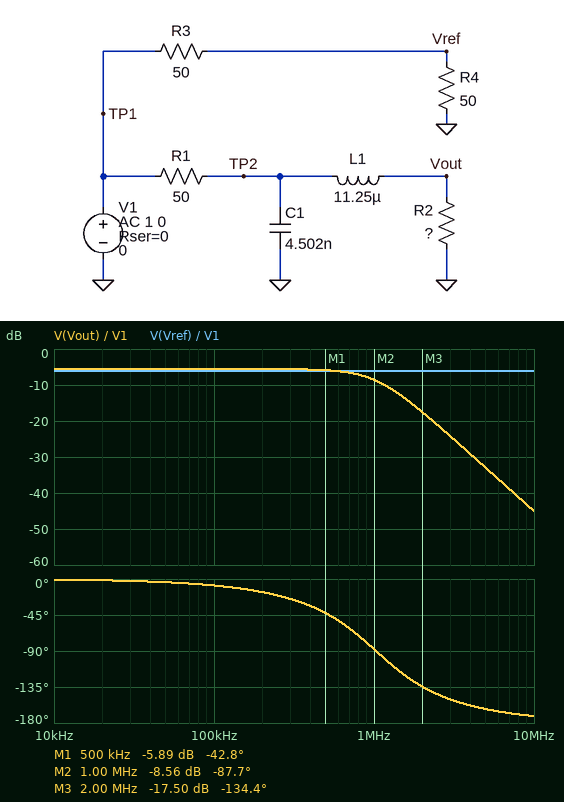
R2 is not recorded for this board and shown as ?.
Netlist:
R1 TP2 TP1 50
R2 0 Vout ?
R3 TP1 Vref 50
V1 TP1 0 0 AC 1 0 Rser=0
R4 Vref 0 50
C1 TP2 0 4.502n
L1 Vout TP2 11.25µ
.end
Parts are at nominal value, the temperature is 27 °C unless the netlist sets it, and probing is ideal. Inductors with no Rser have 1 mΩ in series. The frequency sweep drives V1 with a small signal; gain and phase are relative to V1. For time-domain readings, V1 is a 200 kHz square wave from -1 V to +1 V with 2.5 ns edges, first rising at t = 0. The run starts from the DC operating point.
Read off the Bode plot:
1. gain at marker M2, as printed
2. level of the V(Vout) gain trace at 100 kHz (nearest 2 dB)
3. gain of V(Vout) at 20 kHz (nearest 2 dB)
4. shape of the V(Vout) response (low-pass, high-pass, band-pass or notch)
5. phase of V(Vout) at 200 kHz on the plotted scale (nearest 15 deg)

-8.56 dB
-6 dB
-6 dB
low-pass
-15 deg
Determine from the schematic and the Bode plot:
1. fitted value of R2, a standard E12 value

56 Ω
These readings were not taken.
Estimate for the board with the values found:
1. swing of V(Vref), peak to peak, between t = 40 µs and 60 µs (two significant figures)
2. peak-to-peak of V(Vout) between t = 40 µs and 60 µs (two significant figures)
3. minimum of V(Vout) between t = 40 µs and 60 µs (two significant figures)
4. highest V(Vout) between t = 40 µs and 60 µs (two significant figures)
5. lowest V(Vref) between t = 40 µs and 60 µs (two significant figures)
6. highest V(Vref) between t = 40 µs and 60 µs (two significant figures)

1.0 V
1.1 V
-570 mV
570 mV
-500 mV
500 mV
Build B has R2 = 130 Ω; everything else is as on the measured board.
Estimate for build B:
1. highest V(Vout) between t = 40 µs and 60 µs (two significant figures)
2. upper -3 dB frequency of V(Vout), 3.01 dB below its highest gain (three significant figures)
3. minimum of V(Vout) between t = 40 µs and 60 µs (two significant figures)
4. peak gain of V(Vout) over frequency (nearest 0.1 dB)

720 mV
930 kHz
-720 mV
-2.8 dB
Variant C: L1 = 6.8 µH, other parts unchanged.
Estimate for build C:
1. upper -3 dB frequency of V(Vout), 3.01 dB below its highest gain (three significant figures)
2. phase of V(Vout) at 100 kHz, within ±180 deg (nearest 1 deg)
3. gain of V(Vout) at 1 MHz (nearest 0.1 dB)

1.22 MHz
-7 deg
-7.3 dB
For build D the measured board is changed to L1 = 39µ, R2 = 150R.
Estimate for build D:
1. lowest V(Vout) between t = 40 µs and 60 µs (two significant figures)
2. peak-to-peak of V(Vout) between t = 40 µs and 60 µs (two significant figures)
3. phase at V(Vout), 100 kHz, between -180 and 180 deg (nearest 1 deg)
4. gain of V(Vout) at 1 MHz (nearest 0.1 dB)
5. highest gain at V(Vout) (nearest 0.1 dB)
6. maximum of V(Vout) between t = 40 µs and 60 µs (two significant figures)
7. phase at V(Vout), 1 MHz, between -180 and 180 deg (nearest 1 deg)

-760 mV
1.5 V
-13 deg
-10.1 dB
-2.5 dB
760 mV
-108 deg
